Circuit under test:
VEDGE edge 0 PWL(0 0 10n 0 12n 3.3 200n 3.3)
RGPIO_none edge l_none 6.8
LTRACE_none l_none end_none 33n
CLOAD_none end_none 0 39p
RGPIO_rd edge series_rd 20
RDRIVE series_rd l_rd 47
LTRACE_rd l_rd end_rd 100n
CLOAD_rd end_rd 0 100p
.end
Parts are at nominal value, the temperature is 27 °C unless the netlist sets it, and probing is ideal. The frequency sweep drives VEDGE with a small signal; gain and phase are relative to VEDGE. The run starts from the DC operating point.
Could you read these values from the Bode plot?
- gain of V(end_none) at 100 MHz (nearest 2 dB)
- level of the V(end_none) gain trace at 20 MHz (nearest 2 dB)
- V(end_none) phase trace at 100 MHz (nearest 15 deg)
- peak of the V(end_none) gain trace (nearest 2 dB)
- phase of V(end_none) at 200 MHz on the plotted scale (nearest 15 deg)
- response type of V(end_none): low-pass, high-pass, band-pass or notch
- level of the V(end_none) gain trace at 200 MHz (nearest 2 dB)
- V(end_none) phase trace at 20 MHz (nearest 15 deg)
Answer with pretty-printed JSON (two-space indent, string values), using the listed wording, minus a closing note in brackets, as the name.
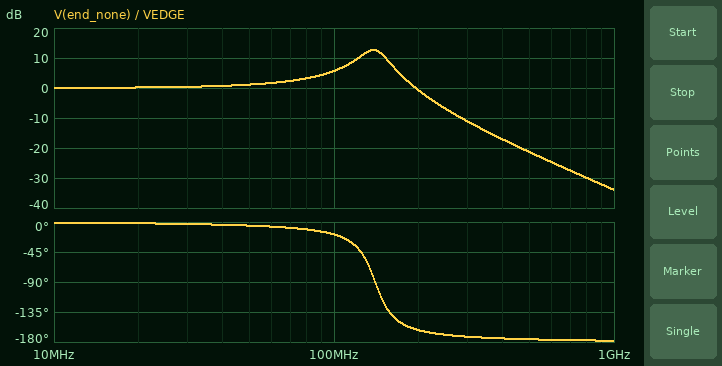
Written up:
{
  "gain of V(end_none) at 100 MHz": "6 dB",
  "level of the V(end_none) gain trace at 20 MHz": "0 dB",
  "V(end_none) phase trace at 100 MHz": "-15 deg",
  "peak of the V(end_none) gain trace": "12 dB",
  "phase of V(end_none) at 200 MHz on the plotted scale": "-165 deg",
  "response type of V(end_none): low-pass, high-pass, band-pass or notch": "low-pass",
  "level of the V(end_none) gain trace at 200 MHz": "0 dB",
  "V(end_none) phase trace at 20 MHz": "0 deg"
}
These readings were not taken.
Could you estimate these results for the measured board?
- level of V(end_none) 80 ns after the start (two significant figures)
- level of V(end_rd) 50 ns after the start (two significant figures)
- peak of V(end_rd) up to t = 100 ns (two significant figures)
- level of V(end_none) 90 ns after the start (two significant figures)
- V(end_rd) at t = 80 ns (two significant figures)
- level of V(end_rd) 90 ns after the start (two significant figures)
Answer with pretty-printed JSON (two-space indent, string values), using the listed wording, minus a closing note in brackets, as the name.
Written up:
{
  "level of V(end_none) 80 ns after the start": "3.3 V",
  "level of V(end_rd) 50 ns after the start": "3.3 V",
  "peak of V(end_rd) up to t = 100 ns": "3.3 V",
  "level of V(end_none) 90 ns after the start": "3.3 V",
  "V(end_rd) at t = 80 ns": "3.3 V",
  "level of V(end_rd) 90 ns after the start": "3.3 V"
}
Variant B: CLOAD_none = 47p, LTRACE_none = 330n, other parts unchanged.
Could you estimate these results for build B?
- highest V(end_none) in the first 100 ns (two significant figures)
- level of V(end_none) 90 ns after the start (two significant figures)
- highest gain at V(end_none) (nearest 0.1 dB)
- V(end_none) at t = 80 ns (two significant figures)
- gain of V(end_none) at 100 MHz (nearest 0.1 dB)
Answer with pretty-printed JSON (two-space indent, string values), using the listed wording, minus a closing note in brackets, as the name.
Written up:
{
  "highest V(end_none) in the first 100 ns": "6.2 V",
  "level of V(end_none) 90 ns after the start": "2.7 V",
  "highest gain at V(end_none)": "21.8 dB",
  "V(end_none) at t = 80 ns": "3.0 V",
  "gain of V(end_none) at 100 MHz": "-14.2 dB"
}
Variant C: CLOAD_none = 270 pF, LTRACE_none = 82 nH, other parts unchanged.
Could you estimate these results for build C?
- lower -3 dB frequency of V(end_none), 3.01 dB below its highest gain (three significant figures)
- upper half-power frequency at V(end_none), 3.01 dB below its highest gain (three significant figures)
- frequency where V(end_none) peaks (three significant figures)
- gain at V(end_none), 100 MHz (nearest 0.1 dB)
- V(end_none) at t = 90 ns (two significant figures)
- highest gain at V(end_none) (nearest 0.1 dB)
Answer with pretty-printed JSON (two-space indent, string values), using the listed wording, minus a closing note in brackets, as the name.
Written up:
{
  "lower -3 dB frequency of V(end_none), 3.01 dB below its highest gain": "24.9 MHz",
  "upper half-power frequency at V(end_none), 3.01 dB below its highest gain": "38.7 MHz",
  "frequency where V(end_none) peaks": "32.5 MHz",
  "gain at V(end_none), 100 MHz": "-17.9 dB",
  "V(end_none) at t = 90 ns": "3.4 V",
  "highest gain at V(end_none)": "8.3 dB"
}
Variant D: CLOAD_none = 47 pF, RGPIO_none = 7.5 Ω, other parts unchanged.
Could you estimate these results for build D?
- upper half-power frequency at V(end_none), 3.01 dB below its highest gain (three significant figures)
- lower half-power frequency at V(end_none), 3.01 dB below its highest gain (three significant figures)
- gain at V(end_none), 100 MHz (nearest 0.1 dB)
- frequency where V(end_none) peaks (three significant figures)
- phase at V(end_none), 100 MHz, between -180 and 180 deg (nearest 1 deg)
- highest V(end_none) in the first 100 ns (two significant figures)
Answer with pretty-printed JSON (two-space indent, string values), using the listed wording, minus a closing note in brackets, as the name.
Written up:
{
  "upper half-power frequency at V(end_none), 3.01 dB below its highest gain": "142 MHz",
  "lower half-power frequency at V(end_none), 3.01 dB below its highest gain": "105 MHz",
  "gain at V(end_none), 100 MHz": "7.0 dB",
  "frequency where V(end_none) peaks": "125 MHz",
  "phase at V(end_none), 100 MHz, between -180 and 180 deg": "-30 deg",
  "highest V(end_none) in the first 100 ns": "5.2 V"
}
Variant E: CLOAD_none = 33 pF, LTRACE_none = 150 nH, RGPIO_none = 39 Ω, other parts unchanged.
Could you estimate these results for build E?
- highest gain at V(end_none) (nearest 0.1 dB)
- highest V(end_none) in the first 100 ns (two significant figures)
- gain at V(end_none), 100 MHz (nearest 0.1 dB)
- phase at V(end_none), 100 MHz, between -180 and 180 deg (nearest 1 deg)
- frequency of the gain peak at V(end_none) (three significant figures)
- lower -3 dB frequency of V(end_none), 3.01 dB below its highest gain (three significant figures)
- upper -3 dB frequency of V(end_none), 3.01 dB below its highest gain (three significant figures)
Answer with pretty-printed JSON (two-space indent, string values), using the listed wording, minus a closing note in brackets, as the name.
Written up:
{
  "highest gain at V(end_none)": "5.1 dB",
  "highest V(end_none) in the first 100 ns": "4.5 V",
  "gain at V(end_none), 100 MHz": "-1.9 dB",
  "phase at V(end_none), 100 MHz, between -180 and 180 deg": "-140 deg",
  "frequency of the gain peak at V(end_none)": "65.3 MHz",
  "lower -3 dB frequency of V(end_none), 3.01 dB below its highest gain": "37.8 MHz",
  "upper -3 dB frequency of V(end_none), 3.01 dB below its highest gain": "84.2 MHz"
}
